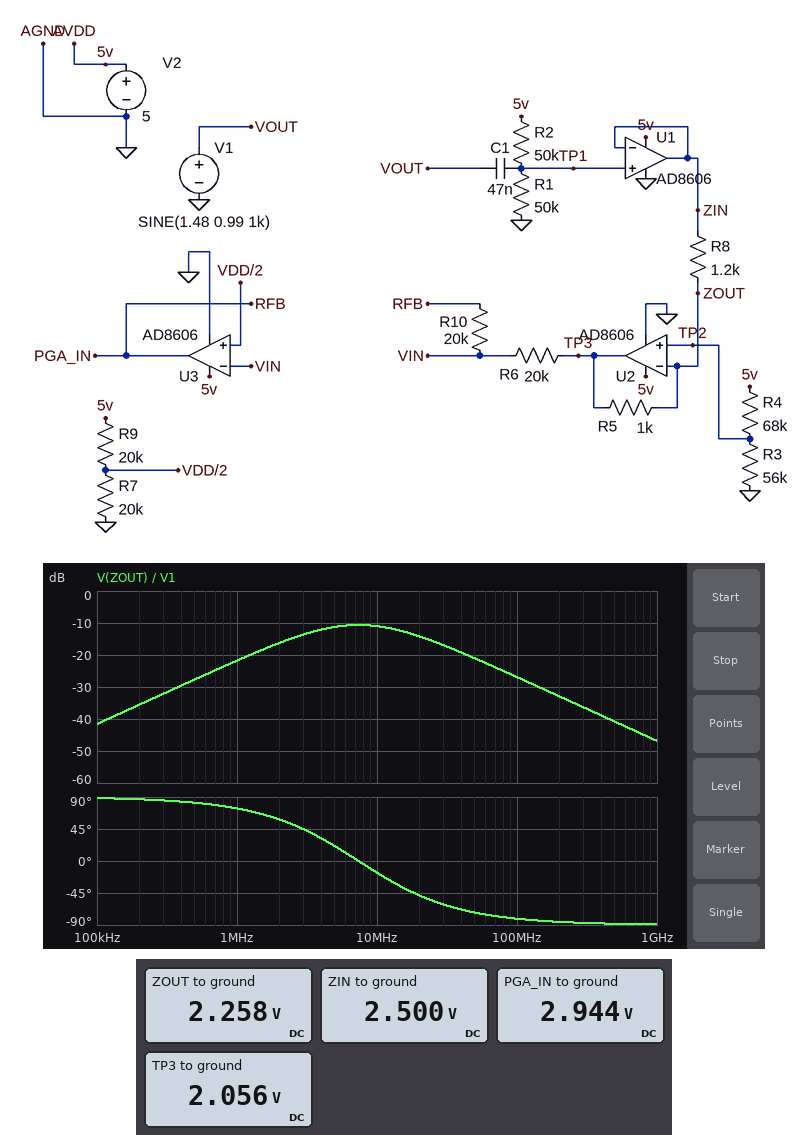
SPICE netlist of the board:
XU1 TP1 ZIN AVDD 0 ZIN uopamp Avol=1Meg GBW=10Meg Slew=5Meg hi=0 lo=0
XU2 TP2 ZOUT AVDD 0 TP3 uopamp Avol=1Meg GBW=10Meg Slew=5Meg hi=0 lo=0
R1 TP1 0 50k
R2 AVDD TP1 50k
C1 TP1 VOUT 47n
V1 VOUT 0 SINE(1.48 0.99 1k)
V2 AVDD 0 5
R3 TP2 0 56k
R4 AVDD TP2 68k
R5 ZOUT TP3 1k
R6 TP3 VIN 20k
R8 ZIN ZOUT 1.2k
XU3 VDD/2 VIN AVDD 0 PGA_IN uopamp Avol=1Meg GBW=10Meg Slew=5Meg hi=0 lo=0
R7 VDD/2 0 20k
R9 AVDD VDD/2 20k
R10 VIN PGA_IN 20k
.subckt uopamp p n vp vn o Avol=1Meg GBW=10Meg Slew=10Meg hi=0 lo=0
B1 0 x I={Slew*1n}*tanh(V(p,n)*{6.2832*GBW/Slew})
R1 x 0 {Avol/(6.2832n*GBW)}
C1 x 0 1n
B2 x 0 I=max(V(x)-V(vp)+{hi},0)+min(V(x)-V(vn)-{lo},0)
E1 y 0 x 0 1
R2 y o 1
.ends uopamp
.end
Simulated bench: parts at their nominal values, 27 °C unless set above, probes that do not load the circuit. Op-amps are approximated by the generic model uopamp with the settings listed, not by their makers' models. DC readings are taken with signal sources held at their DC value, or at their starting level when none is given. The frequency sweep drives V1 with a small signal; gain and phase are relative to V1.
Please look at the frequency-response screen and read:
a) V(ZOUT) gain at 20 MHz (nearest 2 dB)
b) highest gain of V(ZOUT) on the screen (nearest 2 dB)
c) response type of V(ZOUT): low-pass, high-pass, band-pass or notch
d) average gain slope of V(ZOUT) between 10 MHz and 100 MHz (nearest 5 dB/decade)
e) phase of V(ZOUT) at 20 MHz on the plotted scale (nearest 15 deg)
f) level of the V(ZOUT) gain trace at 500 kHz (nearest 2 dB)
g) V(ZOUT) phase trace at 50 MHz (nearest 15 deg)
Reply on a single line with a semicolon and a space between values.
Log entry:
-14 dB; -10 dB; band-pass; -15 dB/decade; -45 deg; -28 dB; -75 deg
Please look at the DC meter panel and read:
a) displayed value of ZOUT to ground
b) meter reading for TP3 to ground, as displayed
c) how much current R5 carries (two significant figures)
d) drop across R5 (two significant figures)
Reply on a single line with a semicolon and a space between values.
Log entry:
2.258 V; 2.056 V; 200 µA; 200 mV
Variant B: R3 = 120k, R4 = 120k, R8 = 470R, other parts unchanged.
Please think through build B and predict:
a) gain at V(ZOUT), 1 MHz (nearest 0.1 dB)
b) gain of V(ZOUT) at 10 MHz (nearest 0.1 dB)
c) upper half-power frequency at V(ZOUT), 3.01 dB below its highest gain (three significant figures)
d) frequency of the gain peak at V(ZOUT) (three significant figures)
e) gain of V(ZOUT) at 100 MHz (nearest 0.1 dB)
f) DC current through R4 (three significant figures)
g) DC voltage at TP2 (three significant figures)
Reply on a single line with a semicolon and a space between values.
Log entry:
-13.9 dB; -6.8 dB; 15.3 MHz; 5.65 MHz; -23.4 dB; 20.8 µA; 2.50 V
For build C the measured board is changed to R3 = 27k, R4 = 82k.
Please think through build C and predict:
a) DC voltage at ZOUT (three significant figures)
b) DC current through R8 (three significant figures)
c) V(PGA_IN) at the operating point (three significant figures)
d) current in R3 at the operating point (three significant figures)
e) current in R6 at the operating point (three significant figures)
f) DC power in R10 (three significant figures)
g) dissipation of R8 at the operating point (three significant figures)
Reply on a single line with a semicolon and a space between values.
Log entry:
1.24 V; 1.05 mA; 4.81 V; 45.9 µA; 116 µA; 267 µW; 1.33 mW
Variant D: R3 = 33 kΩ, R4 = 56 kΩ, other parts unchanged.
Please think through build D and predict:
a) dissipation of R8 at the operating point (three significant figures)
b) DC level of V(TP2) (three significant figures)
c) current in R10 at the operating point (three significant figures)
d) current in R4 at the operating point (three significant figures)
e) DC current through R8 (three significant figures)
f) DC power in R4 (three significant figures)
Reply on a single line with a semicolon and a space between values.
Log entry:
348 µW; 1.85 V; 59.2 µA; 56.2 µA; 538 µA; 177 µW
